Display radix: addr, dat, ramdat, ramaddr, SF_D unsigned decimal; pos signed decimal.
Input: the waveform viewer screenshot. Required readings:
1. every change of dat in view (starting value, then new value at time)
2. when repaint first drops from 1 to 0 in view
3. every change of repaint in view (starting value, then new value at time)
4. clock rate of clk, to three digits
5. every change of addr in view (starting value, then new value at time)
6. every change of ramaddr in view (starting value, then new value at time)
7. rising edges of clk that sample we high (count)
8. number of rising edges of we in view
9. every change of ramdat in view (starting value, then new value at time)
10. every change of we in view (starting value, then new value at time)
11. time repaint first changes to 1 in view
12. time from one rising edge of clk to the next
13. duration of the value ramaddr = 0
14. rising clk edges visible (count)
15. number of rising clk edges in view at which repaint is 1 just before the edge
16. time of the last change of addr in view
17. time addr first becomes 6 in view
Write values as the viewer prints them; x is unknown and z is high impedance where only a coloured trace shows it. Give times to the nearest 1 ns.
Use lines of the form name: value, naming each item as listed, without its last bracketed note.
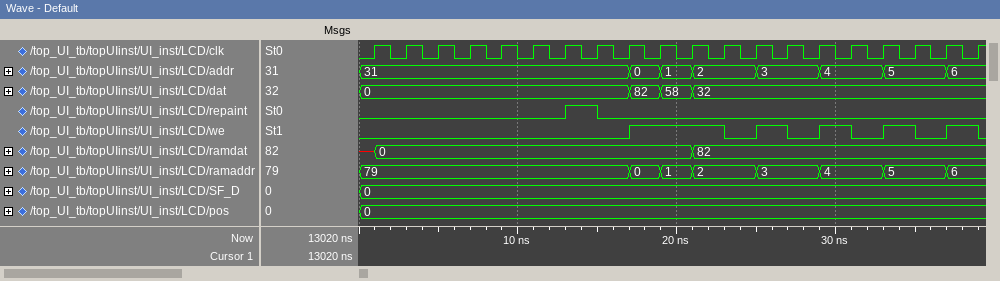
every change of dat in view: 0, 82 at 17 ns, 58 at 19 ns, 32 at 21 ns
when repaint first drops from 1 to 0 in view: 15 ns
every change of repaint in view: 0, 1 at 13 ns, 0 at 15 ns
clock rate of clk, to three digits: 500 MHz
every change of addr in view: 31, 0 at 17 ns, 1 at 19 ns, 2 at 21 ns, 3 at 25 ns, 4 at 29 ns, 5 at 33 ns, 6 at 37 ns
every change of ramaddr in view: 79, 0 at 17 ns, 1 at 19 ns, 2 at 21 ns, 3 at 25 ns, 4 at 29 ns, 5 at 33 ns, 6 at 37 ns
rising edges of clk that sample we high: 7
number of rising edges of we in view: 5
every change of ramdat in view: x, 0 at 1 ns, 82 at 21 ns
every change of we in view: 0, 1 at 17 ns, 0 at 23 ns, 1 at 25 ns, 0 at 27 ns, 1 at 29 ns, 0 at 31 ns, 1 at 33 ns, 0 at 35 ns, 1 at 37 ns, 0 at 39 ns
time repaint first changes to 1 in view: 13 ns
time from one rising edge of clk to the next: 2 ns
duration of the value ramaddr = 0: 2 ns
rising clk edges visible: 20
number of rising clk edges in view at which repaint is 1 just before the edge: 1
time of the last change of addr in view: 37 ns
time addr first becomes 6 in view: 37 ns
